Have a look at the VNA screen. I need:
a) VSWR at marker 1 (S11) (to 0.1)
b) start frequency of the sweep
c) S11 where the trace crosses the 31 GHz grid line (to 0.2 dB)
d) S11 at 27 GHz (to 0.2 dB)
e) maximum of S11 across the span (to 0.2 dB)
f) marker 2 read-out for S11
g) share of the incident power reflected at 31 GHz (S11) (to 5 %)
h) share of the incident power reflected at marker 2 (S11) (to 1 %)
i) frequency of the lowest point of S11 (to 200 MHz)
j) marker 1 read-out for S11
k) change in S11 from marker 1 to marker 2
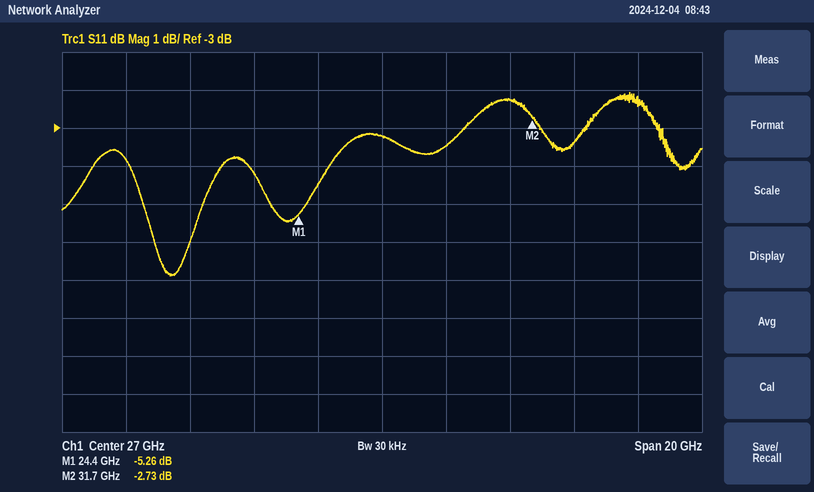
3.4
17 GHz
-2.2 dB
-3.2 dB
-2.0 dB
-2.73 dB
60 %
53 %
20.4 GHz
-5.26 dB
2.53 dB
